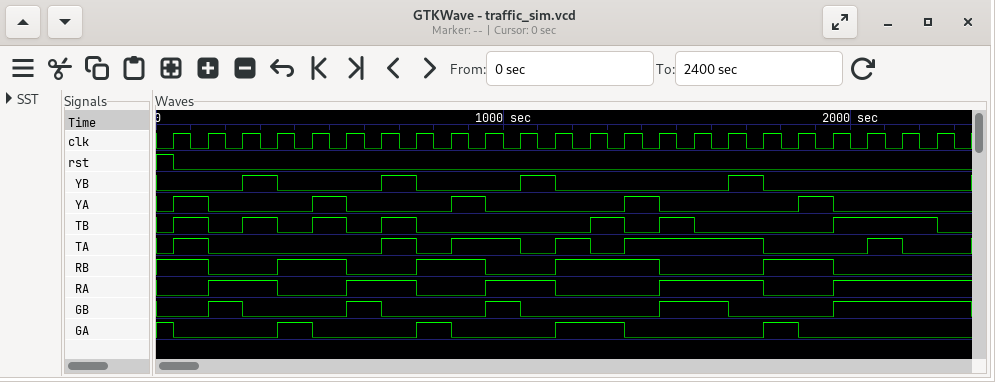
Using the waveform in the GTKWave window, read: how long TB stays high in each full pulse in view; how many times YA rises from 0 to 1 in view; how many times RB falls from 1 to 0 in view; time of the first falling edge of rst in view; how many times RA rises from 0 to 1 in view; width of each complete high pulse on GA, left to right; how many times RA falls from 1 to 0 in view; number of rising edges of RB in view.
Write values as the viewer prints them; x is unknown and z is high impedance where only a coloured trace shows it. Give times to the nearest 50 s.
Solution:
100 s, 100 s, 100 s, 100 s, 100 s, 100 s, 300 s
5
5
50 s
5
100 s, 100 s, 200 s, 100 s
4
4
